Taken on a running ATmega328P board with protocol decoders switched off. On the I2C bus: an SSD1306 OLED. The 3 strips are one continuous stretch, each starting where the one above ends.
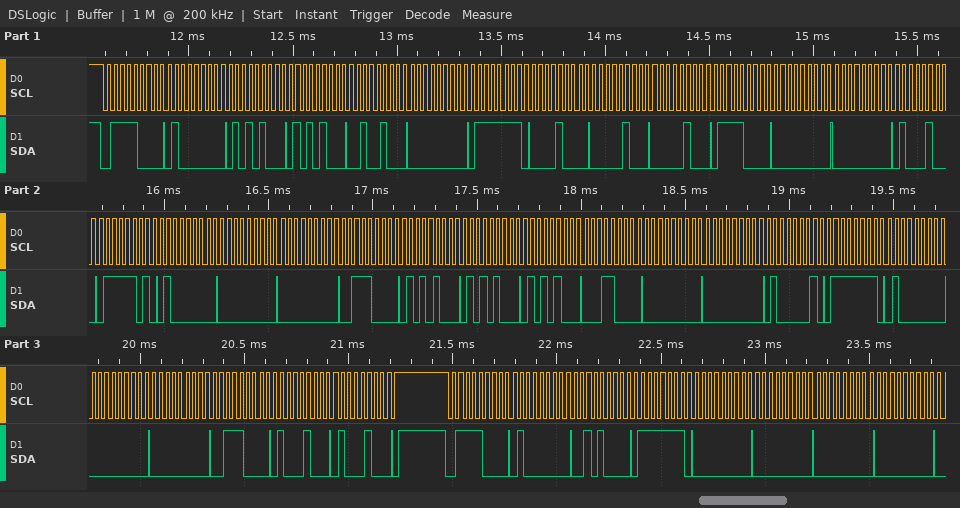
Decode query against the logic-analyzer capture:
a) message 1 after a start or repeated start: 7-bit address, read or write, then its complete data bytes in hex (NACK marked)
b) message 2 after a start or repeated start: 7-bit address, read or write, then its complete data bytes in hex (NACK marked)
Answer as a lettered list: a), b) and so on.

a) 0x3C write: 40 54 54 24 00 7F 08 04 04 78 00 00 44 7D 40 00 00 38 54 54 54 18 00 00 41 7F 40 00 00 38 44 44
b) 0x3C write: 40 28 7F 00 00 00 00
